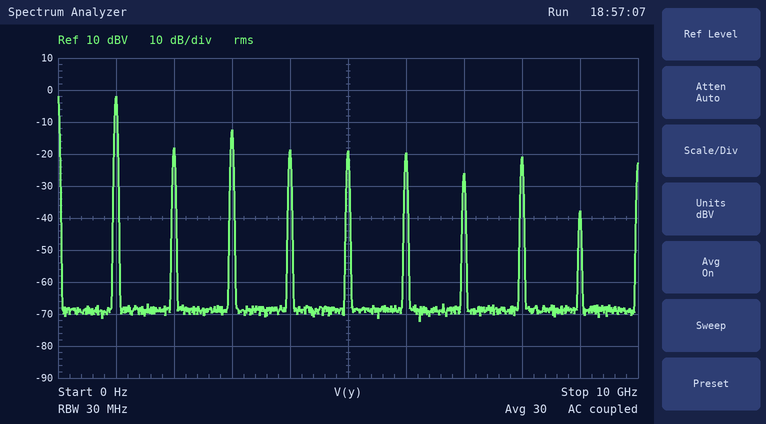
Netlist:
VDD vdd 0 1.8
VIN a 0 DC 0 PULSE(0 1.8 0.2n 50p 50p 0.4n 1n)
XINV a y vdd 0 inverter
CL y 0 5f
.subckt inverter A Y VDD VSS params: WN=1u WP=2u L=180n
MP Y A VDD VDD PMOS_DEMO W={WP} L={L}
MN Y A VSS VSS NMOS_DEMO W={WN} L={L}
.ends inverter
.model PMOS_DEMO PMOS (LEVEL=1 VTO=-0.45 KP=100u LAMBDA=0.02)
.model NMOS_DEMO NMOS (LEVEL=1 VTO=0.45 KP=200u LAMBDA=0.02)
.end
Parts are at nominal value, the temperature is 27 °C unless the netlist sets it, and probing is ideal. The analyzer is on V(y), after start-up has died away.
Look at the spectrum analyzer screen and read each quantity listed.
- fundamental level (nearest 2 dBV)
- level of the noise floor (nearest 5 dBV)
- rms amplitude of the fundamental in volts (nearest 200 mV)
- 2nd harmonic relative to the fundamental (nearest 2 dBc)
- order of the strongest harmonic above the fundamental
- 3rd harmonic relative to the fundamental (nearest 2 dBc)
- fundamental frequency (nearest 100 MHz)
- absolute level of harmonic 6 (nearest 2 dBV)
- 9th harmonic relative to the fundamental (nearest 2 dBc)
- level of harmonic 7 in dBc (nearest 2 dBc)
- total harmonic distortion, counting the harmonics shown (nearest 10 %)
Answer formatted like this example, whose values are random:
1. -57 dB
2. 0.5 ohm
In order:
1. -2 dBV
2. -70 dBV
3. 800 mV
4. -16 dBc
5. 3
6. -10 dBc
7. 1.0 GHz
8. -20 dBV
9. -36 dBc
10. -24 dBc
11. 40 %
